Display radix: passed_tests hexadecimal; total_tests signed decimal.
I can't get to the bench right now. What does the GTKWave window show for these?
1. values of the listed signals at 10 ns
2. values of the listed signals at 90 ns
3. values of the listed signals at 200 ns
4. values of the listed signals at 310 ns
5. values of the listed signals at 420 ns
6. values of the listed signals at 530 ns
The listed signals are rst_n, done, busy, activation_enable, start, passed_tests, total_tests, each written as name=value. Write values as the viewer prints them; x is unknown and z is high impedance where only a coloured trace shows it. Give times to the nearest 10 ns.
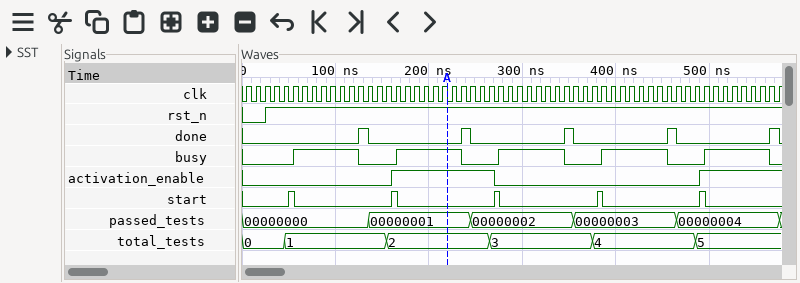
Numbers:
rst_n=0, done=0, busy=0, activation_enable=0, start=0, passed_tests=00000000, total_tests=0
rst_n=1, done=0, busy=1, activation_enable=0, start=0, passed_tests=00000000, total_tests=1
rst_n=1, done=0, busy=1, activation_enable=1, start=0, passed_tests=00000001, total_tests=2
rst_n=1, done=0, busy=1, activation_enable=0, start=0, passed_tests=00000002, total_tests=3
rst_n=1, done=0, busy=1, activation_enable=0, start=0, passed_tests=00000003, total_tests=4
rst_n=1, done=0, busy=1, activation_enable=1, start=0, passed_tests=00000004, total_tests=5
